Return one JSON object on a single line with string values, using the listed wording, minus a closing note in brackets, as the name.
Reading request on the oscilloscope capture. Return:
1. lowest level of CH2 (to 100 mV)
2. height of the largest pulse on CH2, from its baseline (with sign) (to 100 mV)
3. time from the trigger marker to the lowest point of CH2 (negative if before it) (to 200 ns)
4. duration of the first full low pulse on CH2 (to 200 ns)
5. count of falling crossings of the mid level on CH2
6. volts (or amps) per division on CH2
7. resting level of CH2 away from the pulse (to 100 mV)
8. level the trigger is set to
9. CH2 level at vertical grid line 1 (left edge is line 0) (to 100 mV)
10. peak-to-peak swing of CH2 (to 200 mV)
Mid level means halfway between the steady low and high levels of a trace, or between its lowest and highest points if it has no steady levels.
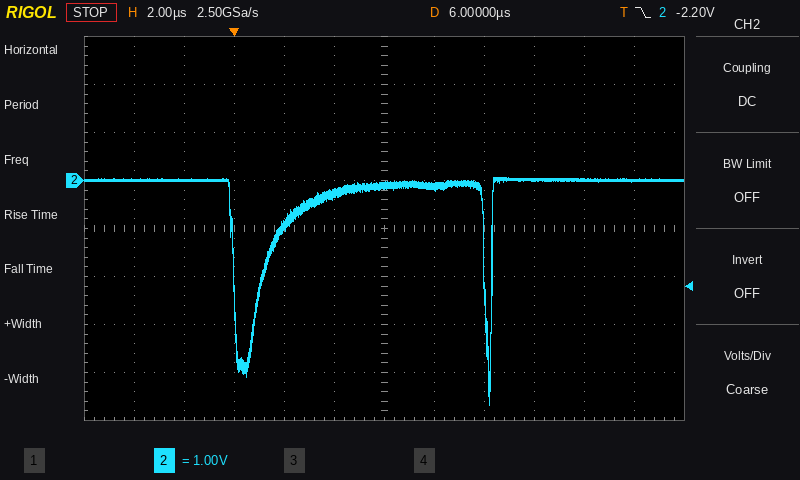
{"lowest level of CH2": "-4.7 V", "height of the largest pulse on CH2, from its baseline (with sign)": "-4.7 V", "time from the trigger marker to the lowest point of CH2 (negative if before it)": "+10.2 µs", "duration of the first full low pulse on CH2": "1.0 µs", "count of falling crossings of the mid level on CH2": "2", "volts (or amps) per division on CH2": "1 V", "resting level of CH2 away from the pulse": "0.0 V", "level the trigger is set to": "-2.20 V", "CH2 level at vertical grid line 1 (left edge is line 0)": "0.0 V", "peak-to-peak swing of CH2": "4.8 V"}
